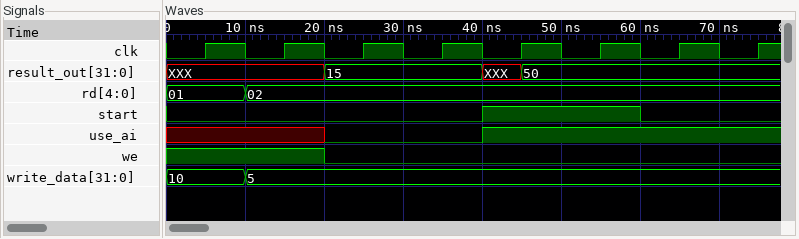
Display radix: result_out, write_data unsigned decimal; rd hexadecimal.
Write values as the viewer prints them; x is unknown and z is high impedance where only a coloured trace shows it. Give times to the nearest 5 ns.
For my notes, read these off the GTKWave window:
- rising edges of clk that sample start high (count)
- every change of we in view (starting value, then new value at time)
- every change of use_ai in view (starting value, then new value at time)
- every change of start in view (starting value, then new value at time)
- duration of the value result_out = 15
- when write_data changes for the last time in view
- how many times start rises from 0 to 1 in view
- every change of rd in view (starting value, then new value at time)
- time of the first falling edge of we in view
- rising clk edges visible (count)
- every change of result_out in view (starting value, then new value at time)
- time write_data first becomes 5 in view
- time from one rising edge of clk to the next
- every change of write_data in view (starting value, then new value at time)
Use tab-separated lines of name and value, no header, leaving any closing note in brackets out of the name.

rising edges of clk that sample start high	2
every change of we in view	1, 0 at 20 ns
every change of use_ai in view	x, 0 at 20 ns, 1 at 40 ns
every change of start in view	0, 1 at 40 ns, 0 at 60 ns
duration of the value result_out = 15	20 ns
when write_data changes for the last time in view	10 ns
how many times start rises from 0 to 1 in view	1
every change of rd in view	01, 02 at 10 ns
time of the first falling edge of we in view	20 ns
rising clk edges visible	8
every change of result_out in view	XXX, 15 at 20 ns, XXX at 40 ns, 50 at 45 ns
time write_data first becomes 5 in view	10 ns
time from one rising edge of clk to the next	10 ns
every change of write_data in view	10, 5 at 10 ns
